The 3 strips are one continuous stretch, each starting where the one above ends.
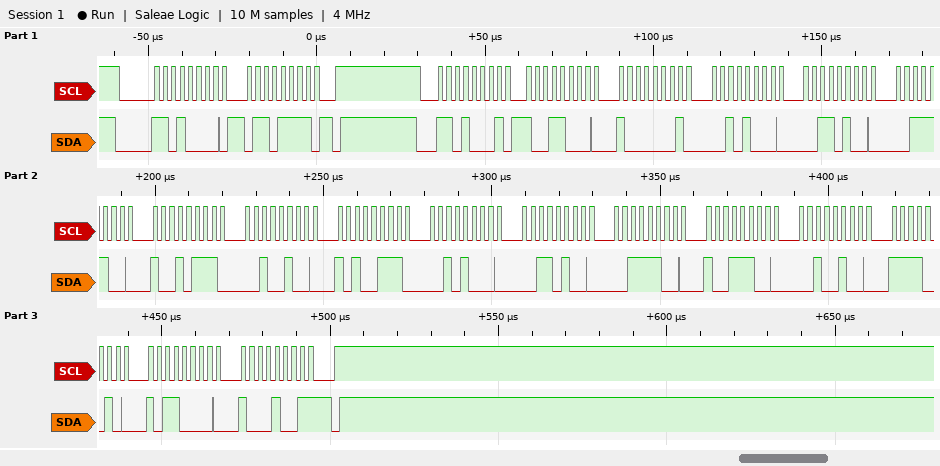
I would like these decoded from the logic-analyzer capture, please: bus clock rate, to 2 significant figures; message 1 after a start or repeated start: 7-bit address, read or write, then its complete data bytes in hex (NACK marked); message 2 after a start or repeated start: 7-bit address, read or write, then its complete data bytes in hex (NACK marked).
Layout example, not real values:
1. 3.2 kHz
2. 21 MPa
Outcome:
1. 400 kHz
2. 0x68 write: 6F
3. 0x68 read: 98 81 28 34 3C 97 24 A7 28 34 3C 9C 24 F2 B0 89 NACK
